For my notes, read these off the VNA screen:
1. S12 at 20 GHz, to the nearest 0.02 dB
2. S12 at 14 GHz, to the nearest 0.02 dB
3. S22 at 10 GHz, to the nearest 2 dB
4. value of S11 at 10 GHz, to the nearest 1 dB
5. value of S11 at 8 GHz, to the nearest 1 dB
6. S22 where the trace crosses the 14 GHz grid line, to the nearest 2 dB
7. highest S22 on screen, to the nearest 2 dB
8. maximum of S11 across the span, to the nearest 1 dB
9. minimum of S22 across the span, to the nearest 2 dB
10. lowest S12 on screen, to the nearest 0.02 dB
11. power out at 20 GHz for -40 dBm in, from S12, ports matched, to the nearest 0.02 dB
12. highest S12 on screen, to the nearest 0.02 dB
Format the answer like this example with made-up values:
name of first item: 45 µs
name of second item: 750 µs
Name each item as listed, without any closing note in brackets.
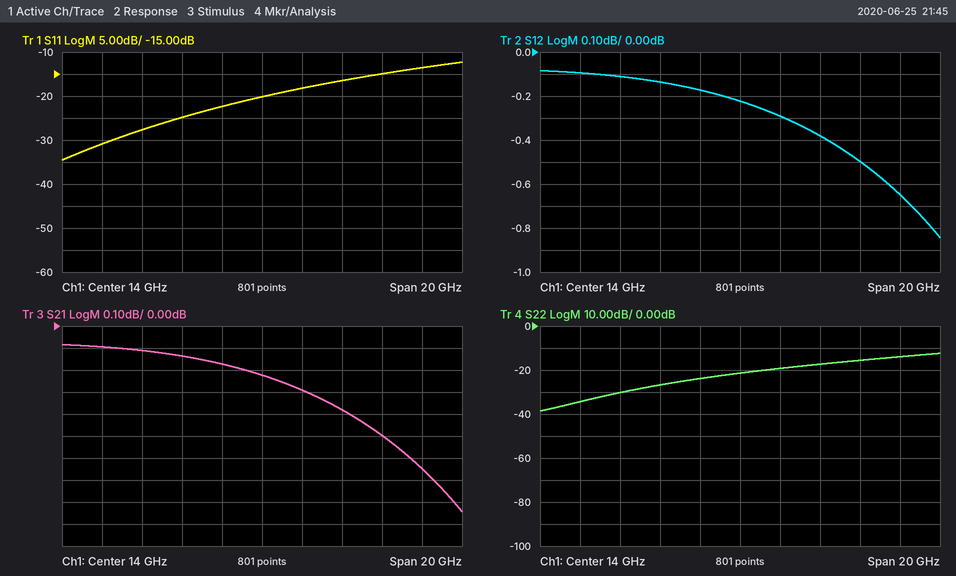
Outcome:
S12 at 20 GHz, to the nearest 0.02 dB: -0.50 dB
S12 at 14 GHz, to the nearest 0.02 dB: -0.22 dB
S22 at 10 GHz, to the nearest 2 dB: -26 dB
value of S11 at 10 GHz, to the nearest 1 dB: -25 dB
value of S11 at 8 GHz, to the nearest 1 dB: -28 dB
S22 where the trace crosses the 14 GHz grid line, to the nearest 2 dB: -22 dB
highest S22 on screen, to the nearest 2 dB: -12 dB
maximum of S11 across the span, to the nearest 1 dB: -12 dB
minimum of S22 across the span, to the nearest 2 dB: -38 dB
lowest S12 on screen, to the nearest 0.02 dB: -0.84 dB
power out at 20 GHz for -40 dBm in, from S12, ports matched, to the nearest 0.02 dB: -40.50 dBm
highest S12 on screen, to the nearest 0.02 dB: -0.08 dB
